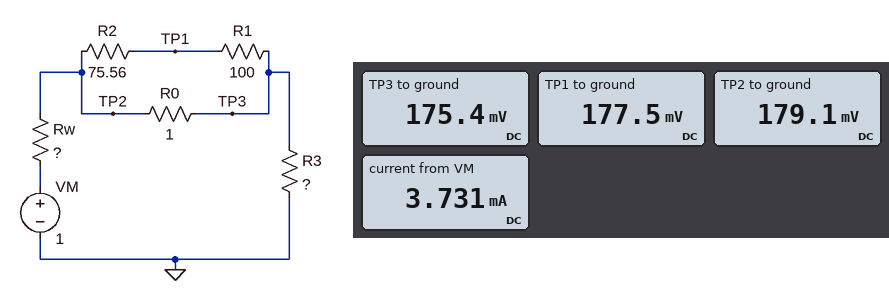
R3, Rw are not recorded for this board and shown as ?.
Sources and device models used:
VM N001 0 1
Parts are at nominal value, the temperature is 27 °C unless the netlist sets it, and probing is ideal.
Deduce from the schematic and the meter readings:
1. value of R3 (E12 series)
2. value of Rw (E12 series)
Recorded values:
47 Ω
220 Ω
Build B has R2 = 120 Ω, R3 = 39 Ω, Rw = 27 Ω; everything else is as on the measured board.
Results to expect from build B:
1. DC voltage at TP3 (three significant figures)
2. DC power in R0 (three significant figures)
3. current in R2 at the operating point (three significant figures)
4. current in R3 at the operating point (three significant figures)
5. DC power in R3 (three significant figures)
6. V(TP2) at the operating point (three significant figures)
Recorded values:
582 mV
221 µW
67.5 µA
14.9 mA
8.69 mW
597 mV
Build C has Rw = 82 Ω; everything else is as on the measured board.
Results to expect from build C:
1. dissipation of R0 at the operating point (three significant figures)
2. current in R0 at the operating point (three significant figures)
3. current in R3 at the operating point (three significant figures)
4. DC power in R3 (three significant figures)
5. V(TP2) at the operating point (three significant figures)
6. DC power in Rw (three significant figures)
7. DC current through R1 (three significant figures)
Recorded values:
58.5 µW
7.65 mA
7.69 mA
2.78 mW
369 mV
4.85 mW
43.6 µA
